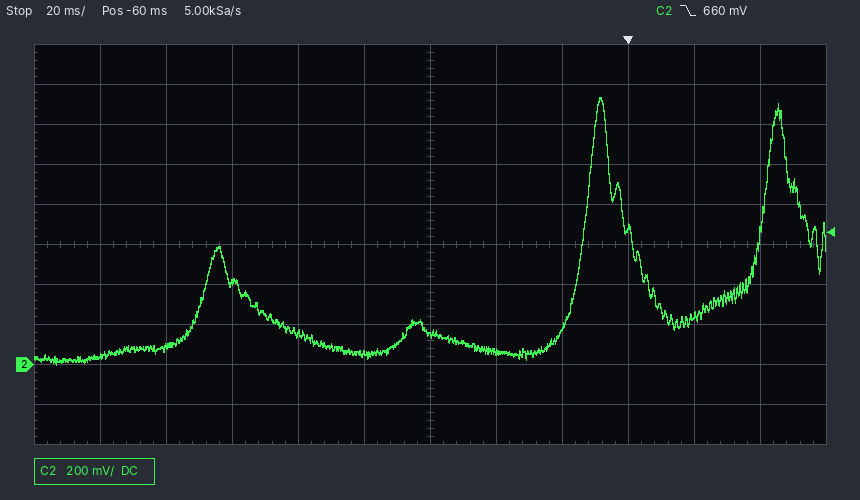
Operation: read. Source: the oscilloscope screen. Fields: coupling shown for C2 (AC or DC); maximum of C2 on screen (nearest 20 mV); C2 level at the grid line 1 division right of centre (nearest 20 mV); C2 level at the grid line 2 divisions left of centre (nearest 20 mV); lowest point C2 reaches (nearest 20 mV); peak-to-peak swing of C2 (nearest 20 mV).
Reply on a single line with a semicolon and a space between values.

DC; 1.34 V; 60 mV; 160 mV; 0 mV; 1.34 V
